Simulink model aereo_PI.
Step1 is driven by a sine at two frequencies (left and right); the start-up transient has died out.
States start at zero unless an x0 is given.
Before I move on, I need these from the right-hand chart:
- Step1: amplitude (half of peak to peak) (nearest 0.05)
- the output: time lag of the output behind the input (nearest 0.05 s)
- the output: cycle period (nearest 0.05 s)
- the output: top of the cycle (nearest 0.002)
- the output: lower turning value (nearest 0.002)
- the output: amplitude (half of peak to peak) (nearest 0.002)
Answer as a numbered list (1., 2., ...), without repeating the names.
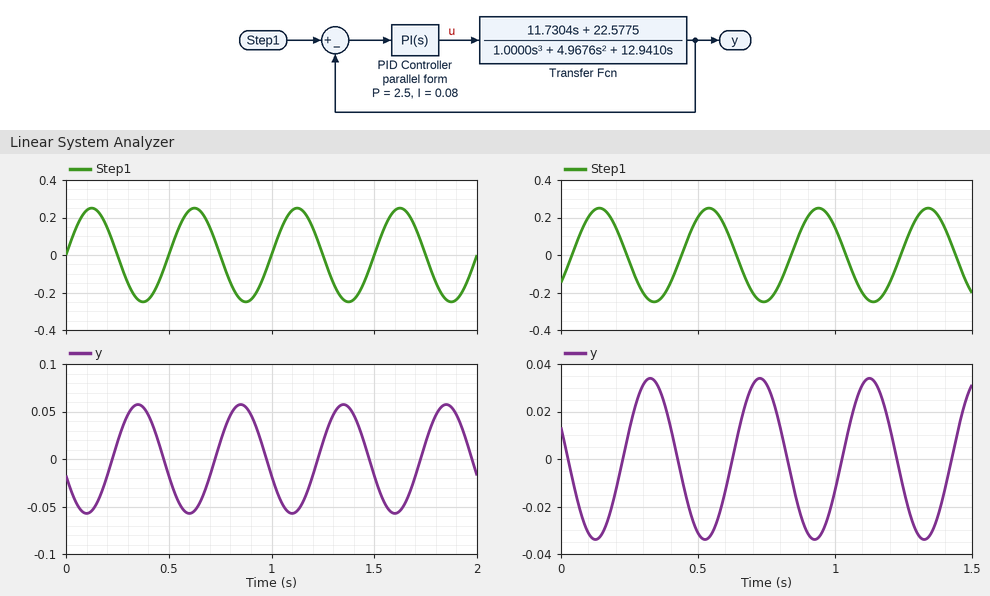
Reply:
1. 0.25
2. 0.20 s
3. 0.40 s
4. 0.034
5. -0.034
6. 0.034
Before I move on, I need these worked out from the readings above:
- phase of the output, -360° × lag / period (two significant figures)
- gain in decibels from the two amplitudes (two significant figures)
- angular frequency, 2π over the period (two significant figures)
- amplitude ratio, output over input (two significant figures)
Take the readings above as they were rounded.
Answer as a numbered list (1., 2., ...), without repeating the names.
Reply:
1. -180°
2. -17 dB
3. 16 rad/s
4. 0.14
